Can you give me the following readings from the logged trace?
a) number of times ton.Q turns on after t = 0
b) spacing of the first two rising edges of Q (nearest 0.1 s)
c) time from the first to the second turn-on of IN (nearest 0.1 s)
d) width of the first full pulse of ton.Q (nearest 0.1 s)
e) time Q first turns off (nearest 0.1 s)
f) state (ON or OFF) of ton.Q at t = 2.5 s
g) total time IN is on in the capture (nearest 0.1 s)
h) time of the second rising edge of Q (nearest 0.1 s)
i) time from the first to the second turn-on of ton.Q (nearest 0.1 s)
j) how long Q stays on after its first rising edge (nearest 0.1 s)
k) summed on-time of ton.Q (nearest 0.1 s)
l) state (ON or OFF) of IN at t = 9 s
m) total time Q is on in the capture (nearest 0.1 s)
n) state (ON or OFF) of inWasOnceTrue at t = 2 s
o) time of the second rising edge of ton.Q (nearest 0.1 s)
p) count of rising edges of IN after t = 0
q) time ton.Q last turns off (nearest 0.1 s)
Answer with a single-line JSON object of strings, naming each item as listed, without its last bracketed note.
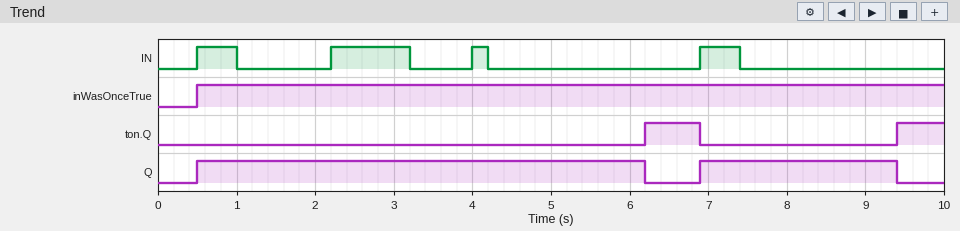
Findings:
{"number of times ton.Q turns on after t = 0": "2", "spacing of the first two rising edges of Q": "6.4 s", "time from the first to the second turn-on of IN": "1.7 s", "width of the first full pulse of ton.Q": "0.7 s", "time Q first turns off": "6.2 s", "state (ON or OFF) of ton.Q at t = 2.5 s": "OFF", "total time IN is on in the capture": "2.2 s", "time of the second rising edge of Q": "6.9 s", "time from the first to the second turn-on of ton.Q": "3.2 s", "how long Q stays on after its first rising edge": "5.7 s", "summed on-time of ton.Q": "1.3 s", "state (ON or OFF) of IN at t = 9 s": "OFF", "total time Q is on in the capture": "8.2 s", "state (ON or OFF) of inWasOnceTrue at t = 2 s": "ON", "time of the second rising edge of ton.Q": "9.4 s", "count of rising edges of IN after t = 0": "4", "time ton.Q last turns off": "6.9 s"}
